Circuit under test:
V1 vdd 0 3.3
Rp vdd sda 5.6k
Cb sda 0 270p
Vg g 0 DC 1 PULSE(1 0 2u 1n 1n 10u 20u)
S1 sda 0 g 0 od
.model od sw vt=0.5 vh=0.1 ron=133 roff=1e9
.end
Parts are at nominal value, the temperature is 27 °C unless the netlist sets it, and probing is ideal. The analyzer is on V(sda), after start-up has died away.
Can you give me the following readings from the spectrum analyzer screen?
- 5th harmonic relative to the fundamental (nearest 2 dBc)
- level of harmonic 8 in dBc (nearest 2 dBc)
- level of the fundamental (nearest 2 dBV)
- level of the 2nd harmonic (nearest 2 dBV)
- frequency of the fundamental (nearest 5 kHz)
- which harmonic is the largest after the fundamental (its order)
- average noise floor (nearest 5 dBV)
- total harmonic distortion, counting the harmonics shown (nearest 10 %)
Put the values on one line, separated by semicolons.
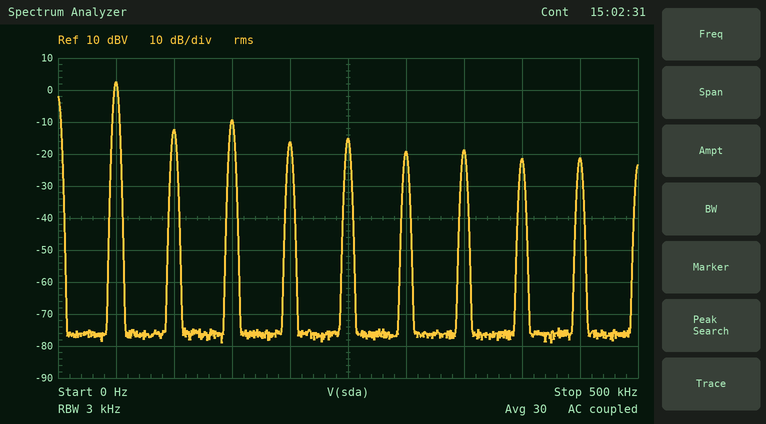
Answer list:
-18 dBc; -24 dBc; 2 dBV; -12 dBV; 50 kHz; 3; -75 dBV; 40 %
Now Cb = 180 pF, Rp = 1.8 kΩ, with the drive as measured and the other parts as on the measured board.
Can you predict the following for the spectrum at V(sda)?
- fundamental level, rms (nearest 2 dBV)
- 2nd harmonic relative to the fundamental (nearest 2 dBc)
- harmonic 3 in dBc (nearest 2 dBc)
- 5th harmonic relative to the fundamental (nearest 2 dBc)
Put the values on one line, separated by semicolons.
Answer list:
2 dBV; -26 dBc; -10 dBc; -14 dBc
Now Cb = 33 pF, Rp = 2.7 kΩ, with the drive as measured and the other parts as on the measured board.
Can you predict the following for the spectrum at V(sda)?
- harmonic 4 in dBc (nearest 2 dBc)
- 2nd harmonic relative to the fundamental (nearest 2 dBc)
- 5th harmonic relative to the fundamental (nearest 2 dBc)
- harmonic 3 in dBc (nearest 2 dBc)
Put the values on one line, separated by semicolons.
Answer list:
-38 dBc; -38 dBc; -14 dBc; -10 dBc
